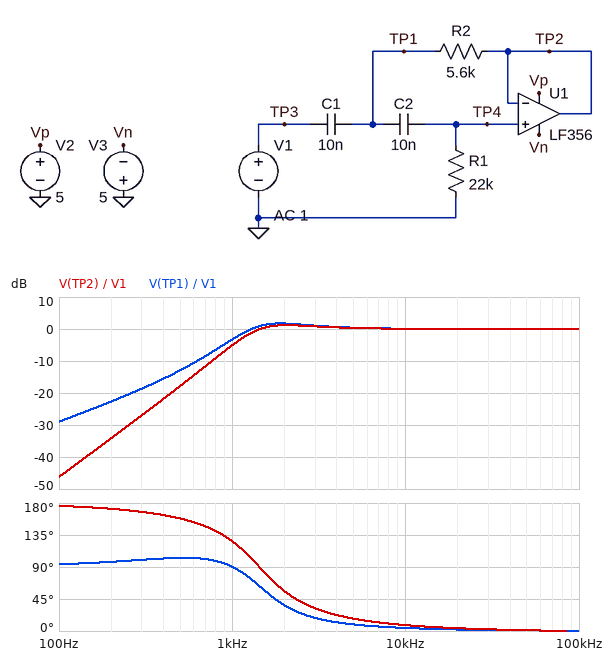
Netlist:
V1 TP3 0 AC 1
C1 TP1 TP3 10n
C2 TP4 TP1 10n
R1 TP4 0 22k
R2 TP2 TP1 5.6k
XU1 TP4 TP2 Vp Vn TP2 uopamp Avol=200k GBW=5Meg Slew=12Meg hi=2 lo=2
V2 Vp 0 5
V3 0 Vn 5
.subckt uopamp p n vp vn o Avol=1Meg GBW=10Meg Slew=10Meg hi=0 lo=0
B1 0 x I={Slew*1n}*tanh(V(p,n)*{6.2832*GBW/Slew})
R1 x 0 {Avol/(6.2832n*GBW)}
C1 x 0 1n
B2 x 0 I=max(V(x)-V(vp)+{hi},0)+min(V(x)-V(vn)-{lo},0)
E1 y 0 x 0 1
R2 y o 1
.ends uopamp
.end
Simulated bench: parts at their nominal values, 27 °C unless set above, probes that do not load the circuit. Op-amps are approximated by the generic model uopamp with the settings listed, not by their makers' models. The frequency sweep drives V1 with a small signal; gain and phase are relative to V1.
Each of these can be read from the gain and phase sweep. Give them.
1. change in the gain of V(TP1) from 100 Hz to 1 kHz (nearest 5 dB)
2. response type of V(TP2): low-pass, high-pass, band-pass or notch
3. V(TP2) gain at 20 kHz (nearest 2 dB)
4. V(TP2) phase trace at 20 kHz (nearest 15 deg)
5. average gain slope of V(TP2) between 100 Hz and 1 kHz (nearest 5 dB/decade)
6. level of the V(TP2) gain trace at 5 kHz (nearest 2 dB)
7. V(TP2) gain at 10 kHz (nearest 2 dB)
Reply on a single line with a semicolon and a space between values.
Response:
25 dB; high-pass; 0 dB; 0 deg; 40 dB/decade; 0 dB; 0 dB
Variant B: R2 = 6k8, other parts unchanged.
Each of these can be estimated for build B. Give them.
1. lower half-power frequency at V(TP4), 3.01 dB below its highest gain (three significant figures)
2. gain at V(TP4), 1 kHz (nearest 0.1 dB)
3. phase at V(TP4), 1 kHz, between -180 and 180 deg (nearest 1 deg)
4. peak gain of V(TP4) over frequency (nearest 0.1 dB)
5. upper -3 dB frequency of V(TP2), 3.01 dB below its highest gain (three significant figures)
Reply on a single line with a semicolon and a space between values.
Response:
1.14 kHz; -4.1 dB; 116 deg; 0.7 dB; 4.21 MHz
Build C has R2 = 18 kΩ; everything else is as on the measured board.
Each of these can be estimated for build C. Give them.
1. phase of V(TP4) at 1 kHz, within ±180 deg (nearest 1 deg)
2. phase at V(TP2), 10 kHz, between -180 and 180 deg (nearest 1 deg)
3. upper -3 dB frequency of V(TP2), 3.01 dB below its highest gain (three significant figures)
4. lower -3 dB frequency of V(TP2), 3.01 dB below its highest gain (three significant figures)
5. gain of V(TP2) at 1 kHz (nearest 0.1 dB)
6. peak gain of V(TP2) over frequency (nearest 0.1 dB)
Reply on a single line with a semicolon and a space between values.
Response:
76 deg; 8 deg; 5.00 MHz; 1.08 kHz; -3.5 dB; 0 dB
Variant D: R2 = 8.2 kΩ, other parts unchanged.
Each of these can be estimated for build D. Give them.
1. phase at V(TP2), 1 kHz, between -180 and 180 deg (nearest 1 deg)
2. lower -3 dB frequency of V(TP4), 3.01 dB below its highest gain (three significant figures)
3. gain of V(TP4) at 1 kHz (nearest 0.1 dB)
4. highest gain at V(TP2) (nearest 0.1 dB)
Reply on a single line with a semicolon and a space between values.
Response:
106 deg; 1.07 kHz; -3.5 dB; 0.3 dB
